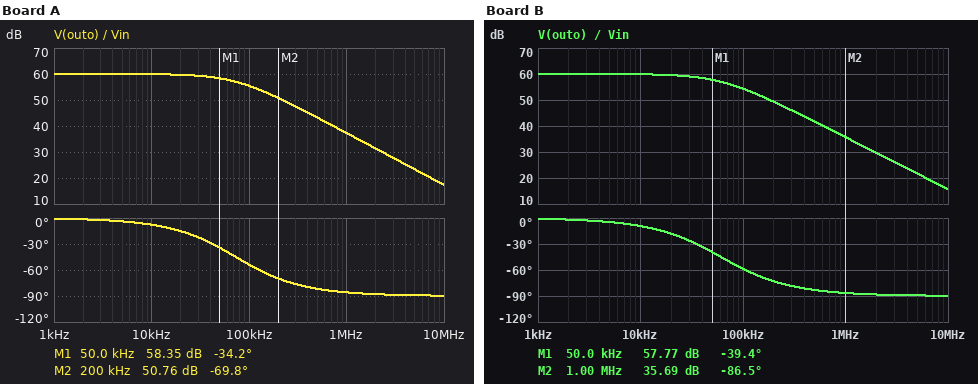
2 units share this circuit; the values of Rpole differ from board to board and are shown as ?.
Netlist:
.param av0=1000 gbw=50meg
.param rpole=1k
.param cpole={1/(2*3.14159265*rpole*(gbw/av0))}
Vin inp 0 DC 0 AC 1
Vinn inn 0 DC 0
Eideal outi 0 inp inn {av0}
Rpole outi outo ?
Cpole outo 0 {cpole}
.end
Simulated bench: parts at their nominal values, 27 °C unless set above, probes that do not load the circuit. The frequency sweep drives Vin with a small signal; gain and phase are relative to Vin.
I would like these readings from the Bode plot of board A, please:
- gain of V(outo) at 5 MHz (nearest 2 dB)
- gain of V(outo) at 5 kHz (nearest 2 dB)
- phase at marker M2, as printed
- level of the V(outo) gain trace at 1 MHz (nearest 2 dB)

24 dB
60 dB
-69.8 deg
38 dB
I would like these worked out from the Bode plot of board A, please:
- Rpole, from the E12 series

680 Ω
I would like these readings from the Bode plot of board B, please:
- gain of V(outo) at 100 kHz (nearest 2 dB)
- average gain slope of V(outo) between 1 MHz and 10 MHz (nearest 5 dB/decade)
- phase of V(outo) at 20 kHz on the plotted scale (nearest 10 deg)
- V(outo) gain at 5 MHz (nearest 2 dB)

54 dB
-20 dB/decade
-20 deg
22 dB
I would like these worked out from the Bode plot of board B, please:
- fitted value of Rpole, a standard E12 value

820 Ω
